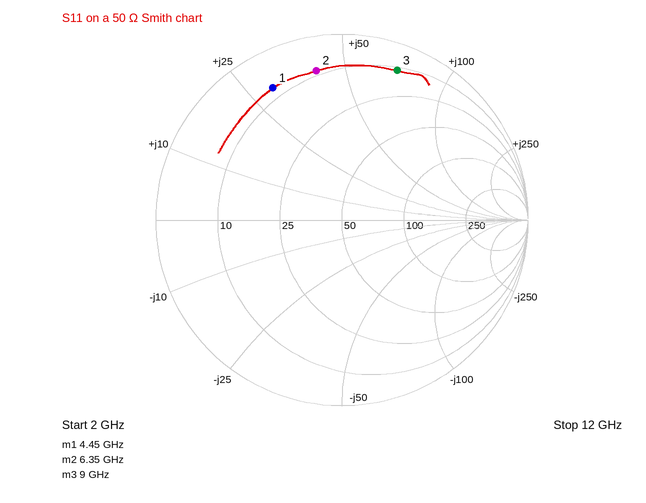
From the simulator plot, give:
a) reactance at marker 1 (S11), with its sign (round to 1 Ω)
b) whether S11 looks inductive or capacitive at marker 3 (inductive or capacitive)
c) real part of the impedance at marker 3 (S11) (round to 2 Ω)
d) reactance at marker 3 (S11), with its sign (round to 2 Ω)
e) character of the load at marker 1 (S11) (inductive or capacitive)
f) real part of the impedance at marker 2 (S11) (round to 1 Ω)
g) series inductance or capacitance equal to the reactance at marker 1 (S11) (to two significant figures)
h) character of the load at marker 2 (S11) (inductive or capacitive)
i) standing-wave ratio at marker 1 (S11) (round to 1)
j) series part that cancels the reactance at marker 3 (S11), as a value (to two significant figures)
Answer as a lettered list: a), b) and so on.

a) +30 Ω
b) inductive
c) 12 Ω
d) +70 Ω
e) inductive
f) 9 Ω
g) 1.1 nH
h) inductive
i) 9
j) 250 fF
